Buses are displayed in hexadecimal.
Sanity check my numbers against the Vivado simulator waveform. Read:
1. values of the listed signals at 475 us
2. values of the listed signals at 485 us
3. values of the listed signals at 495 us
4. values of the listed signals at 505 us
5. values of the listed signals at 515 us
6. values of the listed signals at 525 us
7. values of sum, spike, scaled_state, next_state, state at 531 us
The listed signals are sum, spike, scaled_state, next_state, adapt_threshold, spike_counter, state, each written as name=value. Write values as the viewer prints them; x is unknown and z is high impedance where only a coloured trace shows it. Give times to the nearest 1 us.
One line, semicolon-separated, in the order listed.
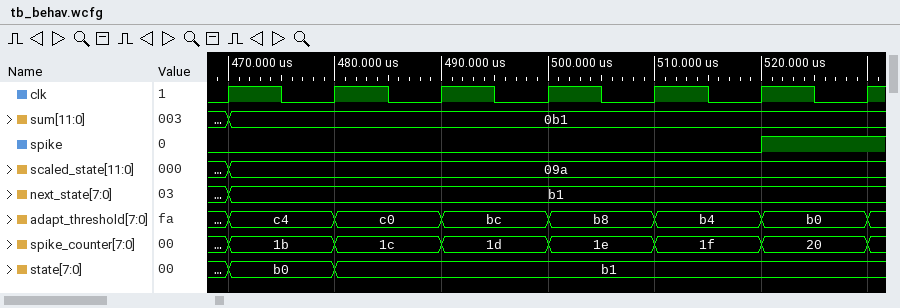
sum=0b1, spike=0, scaled_state=09a, next_state=b1, adapt_threshold=c4, spike_counter=1b, state=b0; sum=0b1, spike=0, scaled_state=09a, next_state=b1, adapt_threshold=c0, spike_counter=1c, state=b1; sum=0b1, spike=0, scaled_state=09a, next_state=b1, adapt_threshold=bc, spike_counter=1d, state=b1; sum=0b1, spike=0, scaled_state=09a, next_state=b1, adapt_threshold=b8, spike_counter=1e, state=b1; sum=0b1, spike=0, scaled_state=09a, next_state=b1, adapt_threshold=b4, spike_counter=1f, state=b1; sum=0b1, spike=1, scaled_state=09a, next_state=b1, adapt_threshold=b0, spike_counter=20, state=b1; sum=0b1, spike=1, scaled_state=09a, next_state=b1, state=b1
